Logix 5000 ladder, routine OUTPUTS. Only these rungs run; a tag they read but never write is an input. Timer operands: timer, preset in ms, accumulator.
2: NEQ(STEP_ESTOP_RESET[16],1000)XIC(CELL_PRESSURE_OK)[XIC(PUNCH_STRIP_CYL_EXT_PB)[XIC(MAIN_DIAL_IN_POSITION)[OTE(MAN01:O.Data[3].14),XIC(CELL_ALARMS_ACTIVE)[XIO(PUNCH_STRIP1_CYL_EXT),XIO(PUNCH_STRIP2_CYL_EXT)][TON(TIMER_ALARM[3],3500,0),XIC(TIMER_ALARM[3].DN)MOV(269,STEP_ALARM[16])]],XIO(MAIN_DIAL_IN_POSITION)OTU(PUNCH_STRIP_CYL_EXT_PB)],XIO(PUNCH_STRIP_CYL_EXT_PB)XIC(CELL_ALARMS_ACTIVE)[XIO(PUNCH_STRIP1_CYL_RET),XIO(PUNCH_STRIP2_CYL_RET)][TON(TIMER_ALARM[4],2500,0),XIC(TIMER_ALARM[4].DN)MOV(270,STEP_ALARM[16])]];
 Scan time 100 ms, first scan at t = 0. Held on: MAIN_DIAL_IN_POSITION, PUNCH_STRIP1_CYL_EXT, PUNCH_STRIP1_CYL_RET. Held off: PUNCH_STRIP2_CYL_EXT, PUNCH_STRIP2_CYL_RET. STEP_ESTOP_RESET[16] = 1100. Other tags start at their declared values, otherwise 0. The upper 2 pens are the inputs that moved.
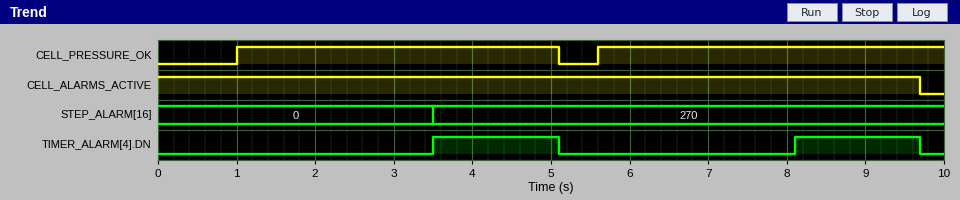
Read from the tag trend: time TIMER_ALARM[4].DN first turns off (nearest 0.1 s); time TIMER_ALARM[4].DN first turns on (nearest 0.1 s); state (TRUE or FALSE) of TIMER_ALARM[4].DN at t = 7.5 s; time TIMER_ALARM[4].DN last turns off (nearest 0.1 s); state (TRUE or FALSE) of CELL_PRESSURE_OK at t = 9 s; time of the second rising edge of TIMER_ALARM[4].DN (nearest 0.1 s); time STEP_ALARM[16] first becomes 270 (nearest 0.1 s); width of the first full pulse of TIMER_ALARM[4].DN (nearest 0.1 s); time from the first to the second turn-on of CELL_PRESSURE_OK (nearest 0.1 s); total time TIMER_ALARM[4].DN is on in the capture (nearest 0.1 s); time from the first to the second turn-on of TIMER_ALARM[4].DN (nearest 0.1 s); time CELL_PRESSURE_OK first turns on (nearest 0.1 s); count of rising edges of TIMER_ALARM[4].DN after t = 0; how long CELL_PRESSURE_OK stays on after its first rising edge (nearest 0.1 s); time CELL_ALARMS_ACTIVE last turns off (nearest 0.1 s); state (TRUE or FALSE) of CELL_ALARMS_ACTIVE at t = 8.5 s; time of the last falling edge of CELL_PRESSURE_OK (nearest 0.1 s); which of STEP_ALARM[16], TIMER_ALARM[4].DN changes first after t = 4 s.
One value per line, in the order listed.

5.1 s
3.5 s
FALSE
9.7 s
TRUE
8.1 s
3.5 s
1.6 s
4.6 s
3.2 s
4.6 s
1.0 s
2
4.1 s
9.7 s
TRUE
5.1 s
TIMER_ALARM[4].DN
